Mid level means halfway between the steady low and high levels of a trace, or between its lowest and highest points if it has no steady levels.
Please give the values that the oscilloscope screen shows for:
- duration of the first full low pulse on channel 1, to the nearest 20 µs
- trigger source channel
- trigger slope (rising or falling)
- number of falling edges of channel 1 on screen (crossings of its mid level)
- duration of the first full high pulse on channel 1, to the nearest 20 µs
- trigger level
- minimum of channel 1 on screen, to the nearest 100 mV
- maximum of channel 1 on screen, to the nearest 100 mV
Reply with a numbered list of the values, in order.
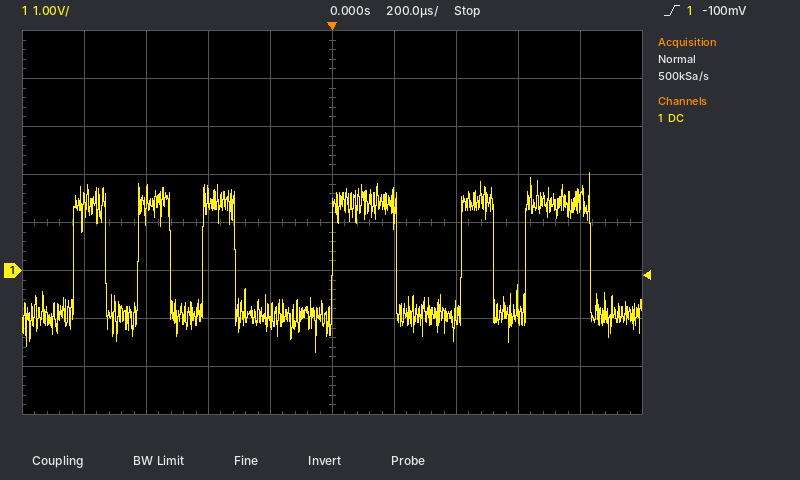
1. 100 µs
2. channel 1
3. rising
4. 6
5. 100 µs
6. -100 mV
7. -1.7 V
8. 2.0 V
